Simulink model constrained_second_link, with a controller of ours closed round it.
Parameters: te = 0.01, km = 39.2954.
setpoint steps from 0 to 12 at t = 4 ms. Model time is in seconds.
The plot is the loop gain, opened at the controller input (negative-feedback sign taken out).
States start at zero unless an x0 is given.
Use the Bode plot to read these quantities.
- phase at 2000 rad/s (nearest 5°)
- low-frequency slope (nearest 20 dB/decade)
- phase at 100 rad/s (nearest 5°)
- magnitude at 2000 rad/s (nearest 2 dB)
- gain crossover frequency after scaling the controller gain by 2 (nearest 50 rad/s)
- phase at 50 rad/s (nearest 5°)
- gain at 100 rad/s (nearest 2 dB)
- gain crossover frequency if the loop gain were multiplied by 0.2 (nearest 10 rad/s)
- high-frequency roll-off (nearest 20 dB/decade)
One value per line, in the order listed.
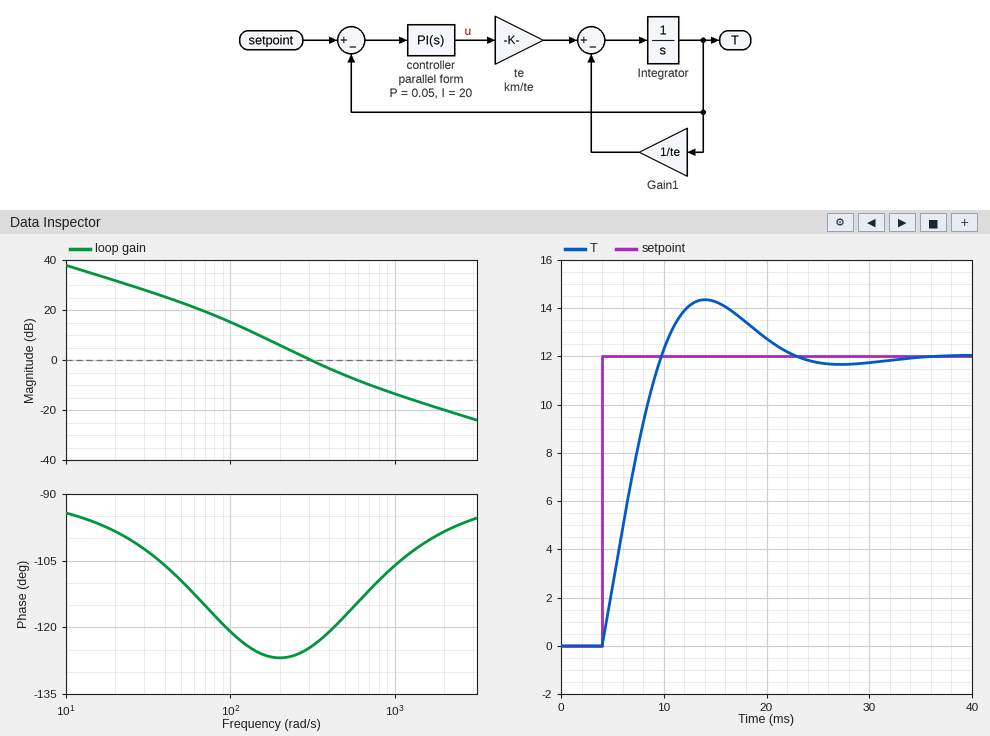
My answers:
-100°
-20 dB/decade
-120°
-20 dB
500 rad/s
-110°
16 dB
110 rad/s
-20 dB/decade
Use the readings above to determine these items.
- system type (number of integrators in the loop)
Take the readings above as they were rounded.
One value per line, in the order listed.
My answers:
1
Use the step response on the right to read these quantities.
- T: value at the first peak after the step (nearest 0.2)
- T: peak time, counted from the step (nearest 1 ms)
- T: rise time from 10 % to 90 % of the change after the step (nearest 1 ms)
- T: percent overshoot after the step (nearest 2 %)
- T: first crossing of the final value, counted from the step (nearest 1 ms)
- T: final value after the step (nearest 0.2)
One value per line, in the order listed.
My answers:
14.4
10 ms
4 ms
20 %
6 ms
12.0
